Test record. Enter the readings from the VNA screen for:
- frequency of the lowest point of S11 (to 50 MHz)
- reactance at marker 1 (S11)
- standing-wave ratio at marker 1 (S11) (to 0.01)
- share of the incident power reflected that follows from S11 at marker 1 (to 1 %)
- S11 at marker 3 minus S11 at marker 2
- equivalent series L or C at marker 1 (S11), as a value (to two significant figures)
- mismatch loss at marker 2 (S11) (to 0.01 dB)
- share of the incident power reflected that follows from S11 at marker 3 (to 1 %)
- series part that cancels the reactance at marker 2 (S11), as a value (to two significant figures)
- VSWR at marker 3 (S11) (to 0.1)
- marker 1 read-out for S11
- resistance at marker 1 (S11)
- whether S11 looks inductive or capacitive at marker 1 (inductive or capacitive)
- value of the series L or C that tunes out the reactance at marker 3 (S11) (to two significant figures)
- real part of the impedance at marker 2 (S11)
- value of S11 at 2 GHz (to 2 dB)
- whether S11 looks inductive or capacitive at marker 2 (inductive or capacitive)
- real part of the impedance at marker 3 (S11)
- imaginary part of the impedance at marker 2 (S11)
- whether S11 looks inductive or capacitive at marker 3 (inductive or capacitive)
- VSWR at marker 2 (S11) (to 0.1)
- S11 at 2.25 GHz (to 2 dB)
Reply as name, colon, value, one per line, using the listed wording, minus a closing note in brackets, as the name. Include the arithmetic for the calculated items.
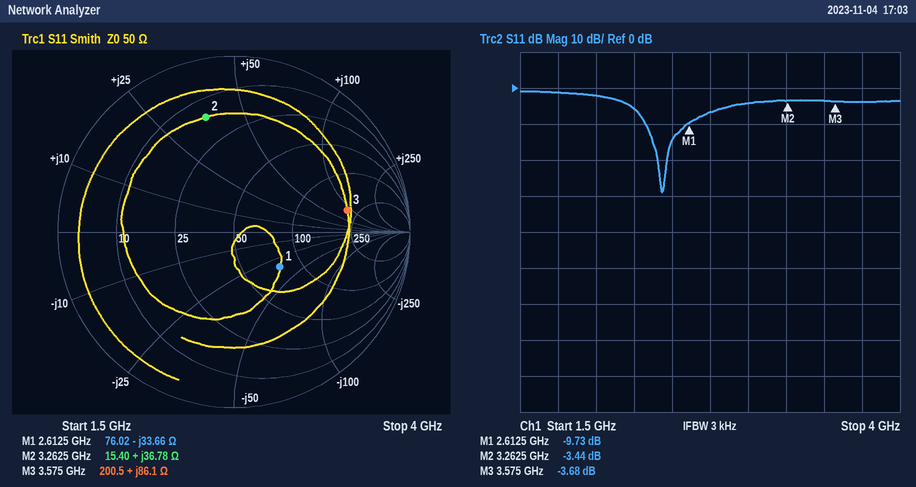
frequency of the lowest point of S11: 2.45 GHz
reactance at marker 1: -33.66 Ω
standing-wave ratio at marker 1 (S11): 1.97
share of the incident power reflected that follows from S11 at marker 1: 10^(-9.73/10) ≈ 11 %
S11 at marker 3 minus S11 at marker 2: -3.68 − (-3.44) = -0.24 dB
equivalent series L or C at marker 1 (S11), as a value: C = 1/(2π × 2.6125 GHz × 33.66 Ω) ≈ 1.8 pF
mismatch loss at marker 2 (S11): −10 log10(1 − 10^(-3.44/10)) ≈ 2.62 dB
share of the incident power reflected that follows from S11 at marker 3: 10^(-3.68/10) ≈ 43 %
series part that cancels the reactance at marker 2 (S11), as a value: C = 1/(2π × 3.2625 GHz × 36.78 Ω) ≈ 1.3 pF
VSWR at marker 3 (S11): 4.8
marker 1 read-out for S11: -9.73 dB
resistance at marker 1: 76.02 Ω
whether S11 looks inductive or capacitive at marker 1: capacitive
value of the series L or C that tunes out the reactance at marker 3 (S11): C = 1/(2π × 3.575 GHz × 86.1 Ω) ≈ 517 fF, so 520 fF to two significant figures
real part of the impedance at marker 2: 15.40 Ω
value of S11 at 2 GHz: -2 dB
whether S11 looks inductive or capacitive at marker 2: inductive
real part of the impedance at marker 3: 200.5 Ω
imaginary part of the impedance at marker 2: +36.78 Ω
whether S11 looks inductive or capacitive at marker 3: inductive
VSWR at marker 2 (S11): 5.1
S11 at 2.25 GHz: -6 dB
